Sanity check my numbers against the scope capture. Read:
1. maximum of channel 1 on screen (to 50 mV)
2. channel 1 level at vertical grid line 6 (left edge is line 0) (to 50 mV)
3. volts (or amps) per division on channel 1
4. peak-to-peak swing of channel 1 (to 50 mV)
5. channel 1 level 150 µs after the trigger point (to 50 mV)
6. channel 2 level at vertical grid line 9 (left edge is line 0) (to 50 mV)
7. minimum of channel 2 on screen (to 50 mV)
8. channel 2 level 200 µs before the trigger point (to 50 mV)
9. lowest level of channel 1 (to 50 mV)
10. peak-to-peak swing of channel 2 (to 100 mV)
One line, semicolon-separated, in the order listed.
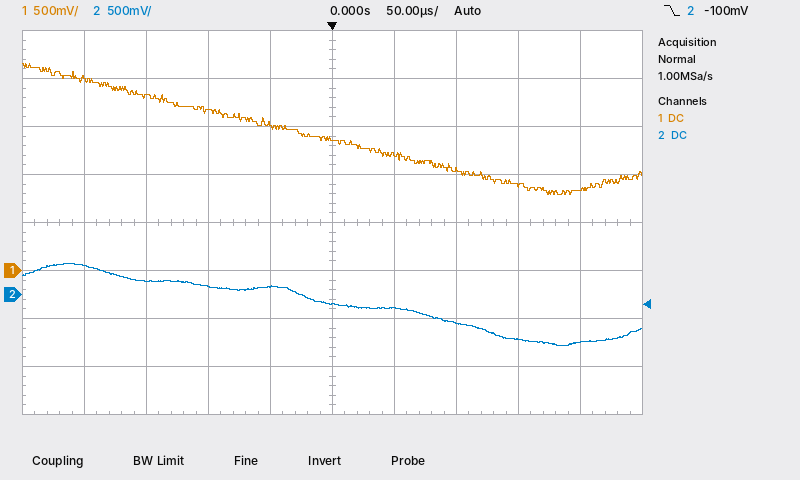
2.15 V; 1.20 V; 500 mV; 1.35 V; 900 mV; -500 mV; -550 mV; 300 mV; 800 mV; 900 mV
